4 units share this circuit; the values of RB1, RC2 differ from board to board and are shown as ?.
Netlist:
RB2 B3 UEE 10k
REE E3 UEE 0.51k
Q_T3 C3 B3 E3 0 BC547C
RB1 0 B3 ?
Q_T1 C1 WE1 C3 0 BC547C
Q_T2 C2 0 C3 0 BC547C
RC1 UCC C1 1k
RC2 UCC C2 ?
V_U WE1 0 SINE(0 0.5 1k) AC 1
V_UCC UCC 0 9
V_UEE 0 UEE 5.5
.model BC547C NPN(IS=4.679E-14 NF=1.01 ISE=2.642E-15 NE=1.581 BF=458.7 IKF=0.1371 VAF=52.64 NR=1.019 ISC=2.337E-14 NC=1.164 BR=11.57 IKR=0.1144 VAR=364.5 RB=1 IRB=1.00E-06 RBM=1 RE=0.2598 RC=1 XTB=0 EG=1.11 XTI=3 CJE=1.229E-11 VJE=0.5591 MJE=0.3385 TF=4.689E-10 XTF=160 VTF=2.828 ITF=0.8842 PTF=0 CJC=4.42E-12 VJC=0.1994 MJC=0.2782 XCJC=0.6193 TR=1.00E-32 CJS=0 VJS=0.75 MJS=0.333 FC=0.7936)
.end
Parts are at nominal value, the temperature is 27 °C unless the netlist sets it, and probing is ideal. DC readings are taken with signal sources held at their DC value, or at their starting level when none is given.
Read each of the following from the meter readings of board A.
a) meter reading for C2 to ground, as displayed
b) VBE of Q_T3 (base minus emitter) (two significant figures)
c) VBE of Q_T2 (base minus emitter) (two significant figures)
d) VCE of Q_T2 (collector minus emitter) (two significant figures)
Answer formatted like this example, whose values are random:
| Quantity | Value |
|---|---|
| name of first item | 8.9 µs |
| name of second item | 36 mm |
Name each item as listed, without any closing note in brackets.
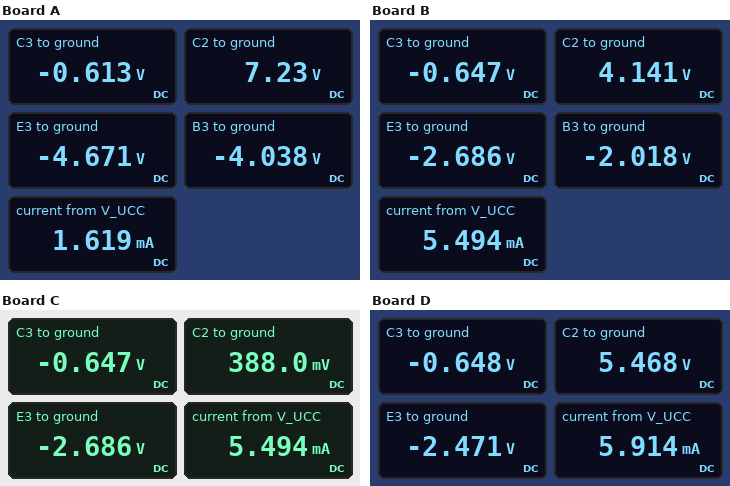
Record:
| Quantity | Value |
|---|---|
| meter reading for C2 to ground, as displayed | 7.23 V |
| VBE of Q_T3 (base minus emitter) | 630 mV |
| VBE of Q_T2 (base minus emitter) | 610 mV |
| VCE of Q_T2 (collector minus emitter) | 7.8 V |
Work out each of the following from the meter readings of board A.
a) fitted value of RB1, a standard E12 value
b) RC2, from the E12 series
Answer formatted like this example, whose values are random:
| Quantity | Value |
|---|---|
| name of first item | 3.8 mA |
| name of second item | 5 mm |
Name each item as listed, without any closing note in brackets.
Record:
| Quantity | Value |
|---|---|
| fitted value of RB1, a standard E12 value | 27 kΩ |
| RC2, from the E12 series | 2.2 kΩ |
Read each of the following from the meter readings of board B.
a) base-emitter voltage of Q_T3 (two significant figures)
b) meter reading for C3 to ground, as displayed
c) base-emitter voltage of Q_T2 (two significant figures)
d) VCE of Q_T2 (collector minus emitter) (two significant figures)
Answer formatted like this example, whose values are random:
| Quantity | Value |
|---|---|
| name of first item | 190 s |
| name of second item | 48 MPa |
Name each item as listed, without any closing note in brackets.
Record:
| Quantity | Value |
|---|---|
| base-emitter voltage of Q_T3 | 670 mV |
| meter reading for C3 to ground, as displayed | -0.647 V |
| base-emitter voltage of Q_T2 | 650 mV |
| VCE of Q_T2 (collector minus emitter) | 4.8 V |
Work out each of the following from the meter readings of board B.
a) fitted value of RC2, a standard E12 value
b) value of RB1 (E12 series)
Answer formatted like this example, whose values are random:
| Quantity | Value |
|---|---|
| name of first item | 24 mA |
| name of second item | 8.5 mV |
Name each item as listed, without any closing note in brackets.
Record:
| Quantity | Value |
|---|---|
| fitted value of RC2, a standard E12 value | 1.8 kΩ |
| value of RB1 | 5.6 kΩ |
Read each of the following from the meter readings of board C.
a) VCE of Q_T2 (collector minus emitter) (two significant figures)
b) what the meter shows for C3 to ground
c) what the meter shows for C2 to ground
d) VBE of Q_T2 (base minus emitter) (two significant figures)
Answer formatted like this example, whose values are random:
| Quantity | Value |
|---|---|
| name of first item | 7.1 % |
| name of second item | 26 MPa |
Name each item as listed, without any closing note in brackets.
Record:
| Quantity | Value |
|---|---|
| VCE of Q_T2 (collector minus emitter) | 1.0 V |
| what the meter shows for C3 to ground | -0.647 V |
| what the meter shows for C2 to ground | 388.0 mV |
| VBE of Q_T2 (base minus emitter) | 650 mV |
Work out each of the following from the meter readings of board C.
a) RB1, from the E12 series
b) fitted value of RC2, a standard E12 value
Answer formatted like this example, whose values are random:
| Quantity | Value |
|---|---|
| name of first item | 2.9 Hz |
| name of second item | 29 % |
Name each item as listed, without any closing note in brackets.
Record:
| Quantity | Value |
|---|---|
| RB1, from the E12 series | 5.6 kΩ |
| fitted value of RC2, a standard E12 value | 3.3 kΩ |
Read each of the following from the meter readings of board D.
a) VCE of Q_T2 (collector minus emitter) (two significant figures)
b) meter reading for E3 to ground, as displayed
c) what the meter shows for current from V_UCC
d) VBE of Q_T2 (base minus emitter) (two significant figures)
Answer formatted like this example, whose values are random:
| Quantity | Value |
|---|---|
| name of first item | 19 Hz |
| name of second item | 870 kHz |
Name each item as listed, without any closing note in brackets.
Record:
| Quantity | Value |
|---|---|
| VCE of Q_T2 (collector minus emitter) | 6.1 V |
| meter reading for E3 to ground, as displayed | -2.471 V |
| what the meter shows for current from V_UCC | 5.914 mA |
| VBE of Q_T2 (base minus emitter) | 650 mV |
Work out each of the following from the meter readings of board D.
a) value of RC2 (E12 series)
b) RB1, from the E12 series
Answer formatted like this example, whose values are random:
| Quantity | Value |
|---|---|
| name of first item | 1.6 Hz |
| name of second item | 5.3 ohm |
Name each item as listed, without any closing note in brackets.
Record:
| Quantity | Value |
|---|---|
| value of RC2 | 1.2 kΩ |
| RB1, from the E12 series | 4.7 kΩ |
